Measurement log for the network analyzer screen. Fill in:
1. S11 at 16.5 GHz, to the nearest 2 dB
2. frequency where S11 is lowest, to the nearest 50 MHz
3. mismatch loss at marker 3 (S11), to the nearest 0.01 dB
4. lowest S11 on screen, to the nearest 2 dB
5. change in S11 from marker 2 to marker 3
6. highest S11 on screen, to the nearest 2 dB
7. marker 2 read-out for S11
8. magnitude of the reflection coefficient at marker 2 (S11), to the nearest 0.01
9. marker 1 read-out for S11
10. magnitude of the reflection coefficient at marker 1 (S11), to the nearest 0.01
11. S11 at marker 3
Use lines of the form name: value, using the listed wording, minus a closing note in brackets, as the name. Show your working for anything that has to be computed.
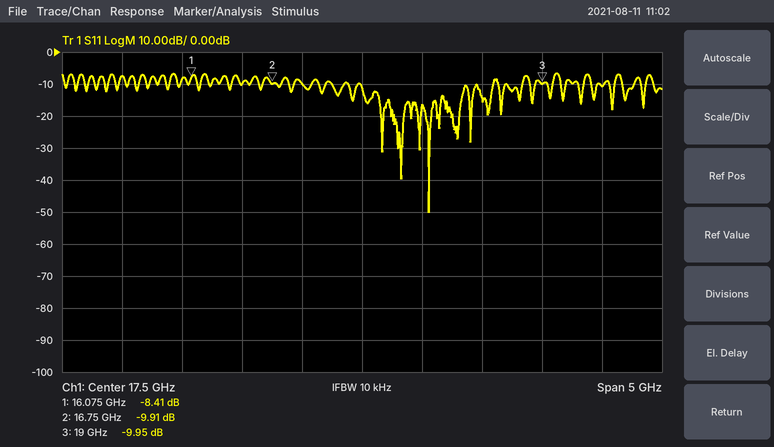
S11 at 16.5 GHz, to the nearest 2 dB: -10 dB
frequency where S11 is lowest, to the nearest 50 MHz: 18.05 GHz
mismatch loss at marker 3 (S11), to the nearest 0.01 dB: −10 log10(1 − 10^(-9.95/10)) ≈ 0.46 dB
lowest S11 on screen, to the nearest 2 dB: -50 dB
change in S11 from marker 2 to marker 3: -9.95 − (-9.91) = -0.04 dB
highest S11 on screen, to the nearest 2 dB: -6 dB
marker 2 read-out for S11: -9.91 dB
magnitude of the reflection coefficient at marker 2 (S11), to the nearest 0.01: 10^(-9.91/20) ≈ 0.32
marker 1 read-out for S11: -8.41 dB
magnitude of the reflection coefficient at marker 1 (S11), to the nearest 0.01: 10^(-8.41/20) ≈ 0.38
S11 at marker 3: -9.95 dB
